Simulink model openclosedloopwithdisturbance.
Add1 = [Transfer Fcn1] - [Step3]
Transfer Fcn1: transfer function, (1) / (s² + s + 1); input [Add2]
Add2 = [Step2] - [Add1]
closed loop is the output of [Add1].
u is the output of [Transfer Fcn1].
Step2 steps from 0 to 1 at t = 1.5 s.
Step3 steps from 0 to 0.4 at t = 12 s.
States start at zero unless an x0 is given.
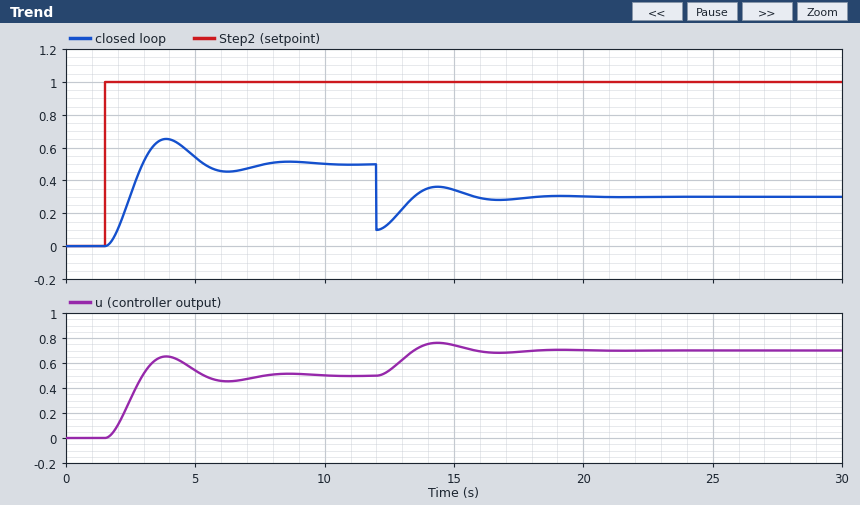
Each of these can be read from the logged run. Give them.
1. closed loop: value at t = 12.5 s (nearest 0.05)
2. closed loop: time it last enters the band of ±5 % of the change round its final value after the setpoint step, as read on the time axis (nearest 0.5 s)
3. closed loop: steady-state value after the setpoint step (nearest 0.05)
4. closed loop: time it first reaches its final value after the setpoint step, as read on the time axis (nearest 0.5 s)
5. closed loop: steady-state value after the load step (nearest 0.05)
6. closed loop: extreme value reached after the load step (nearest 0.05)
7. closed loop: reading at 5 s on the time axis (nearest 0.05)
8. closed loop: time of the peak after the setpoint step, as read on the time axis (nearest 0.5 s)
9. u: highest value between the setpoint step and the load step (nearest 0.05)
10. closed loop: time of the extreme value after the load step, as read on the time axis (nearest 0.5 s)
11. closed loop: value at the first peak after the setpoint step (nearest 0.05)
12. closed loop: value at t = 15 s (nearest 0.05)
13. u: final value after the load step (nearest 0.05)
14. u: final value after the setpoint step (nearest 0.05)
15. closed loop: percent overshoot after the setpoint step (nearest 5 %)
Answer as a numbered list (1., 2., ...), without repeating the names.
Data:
1. 0.15
2. 7.0 s
3. 0.50
4. 3.0 s
5. 0.30
6. 0.10
7. 0.55
8. 4.0 s
9. 0.65
10. 12.0 s
11. 0.65
12. 0.35
13. 0.70
14. 0.50
15. 30 %
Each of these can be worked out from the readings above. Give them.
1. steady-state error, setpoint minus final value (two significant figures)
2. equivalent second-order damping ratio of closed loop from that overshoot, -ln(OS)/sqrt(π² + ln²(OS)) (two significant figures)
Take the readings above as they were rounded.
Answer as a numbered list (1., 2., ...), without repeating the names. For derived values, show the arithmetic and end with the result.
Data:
1. 1 - 0.5 = 0.50
2. ln(0.3) = -1.204; 1.204 / sqrt(9.870 + 1.450) = 0.36
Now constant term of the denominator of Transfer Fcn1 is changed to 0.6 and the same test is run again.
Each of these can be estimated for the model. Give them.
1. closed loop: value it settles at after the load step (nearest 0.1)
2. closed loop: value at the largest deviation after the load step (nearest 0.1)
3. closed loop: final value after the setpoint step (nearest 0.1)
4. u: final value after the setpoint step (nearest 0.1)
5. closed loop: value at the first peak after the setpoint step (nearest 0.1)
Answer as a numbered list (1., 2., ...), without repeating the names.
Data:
1. 0.5
2. 0.2
3. 0.6
4. 0.6
5. 0.8
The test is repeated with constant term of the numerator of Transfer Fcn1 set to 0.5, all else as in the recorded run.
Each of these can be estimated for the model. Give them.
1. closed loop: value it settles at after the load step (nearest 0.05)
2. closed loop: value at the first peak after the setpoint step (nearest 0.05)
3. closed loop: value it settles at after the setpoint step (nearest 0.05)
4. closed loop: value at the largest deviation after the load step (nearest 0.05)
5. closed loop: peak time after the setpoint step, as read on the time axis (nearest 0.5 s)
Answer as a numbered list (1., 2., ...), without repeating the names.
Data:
1. 0.05
2. 0.40
3. 0.35
4. -0.05
5. 4.5 s
